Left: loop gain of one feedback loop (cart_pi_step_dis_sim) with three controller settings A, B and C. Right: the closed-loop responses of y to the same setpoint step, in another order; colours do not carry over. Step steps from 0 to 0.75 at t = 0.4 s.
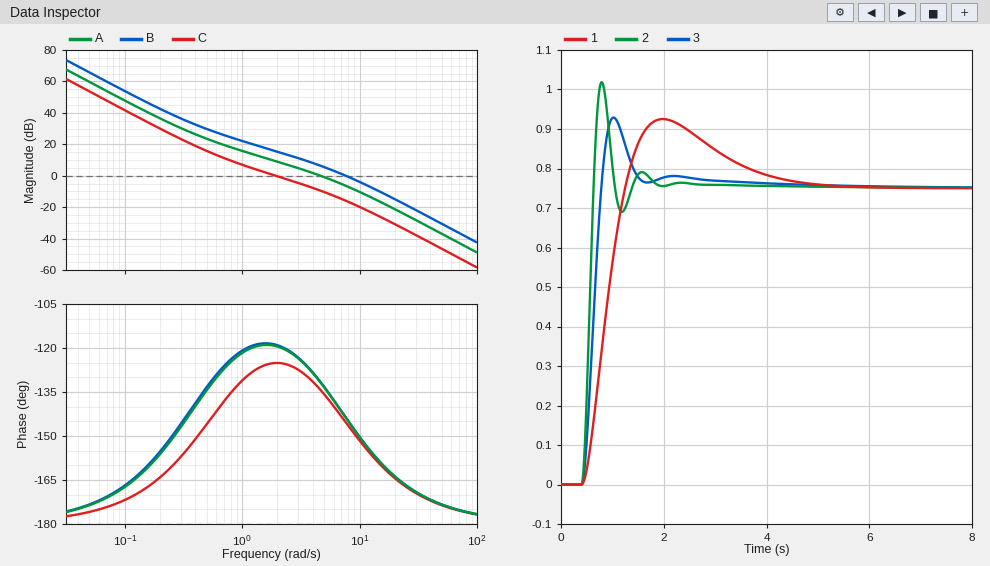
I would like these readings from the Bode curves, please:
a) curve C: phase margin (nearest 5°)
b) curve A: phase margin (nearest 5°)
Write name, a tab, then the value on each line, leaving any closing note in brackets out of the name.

curve C: phase margin	55°
curve A: phase margin	50°
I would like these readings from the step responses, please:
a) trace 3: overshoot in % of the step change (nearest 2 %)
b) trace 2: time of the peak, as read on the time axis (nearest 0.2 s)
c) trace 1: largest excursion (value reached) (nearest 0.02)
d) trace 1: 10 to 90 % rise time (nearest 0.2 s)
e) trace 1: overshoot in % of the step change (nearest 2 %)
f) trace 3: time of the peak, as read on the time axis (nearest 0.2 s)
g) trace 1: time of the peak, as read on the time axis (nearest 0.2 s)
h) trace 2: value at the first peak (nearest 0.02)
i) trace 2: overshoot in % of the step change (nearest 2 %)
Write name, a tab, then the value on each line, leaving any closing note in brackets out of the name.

trace 3: overshoot in % of the step change	24 %
trace 2: time of the peak, as read on the time axis	0.8 s
trace 1: largest excursion (value reached)	0.92
trace 1: 10 to 90 % rise time	0.6 s
trace 1: overshoot in % of the step change	24 %
trace 3: time of the peak, as read on the time axis	1.0 s
trace 1: time of the peak, as read on the time axis	2.0 s
trace 2: value at the first peak	1.02
trace 2: overshoot in % of the step change	36 %
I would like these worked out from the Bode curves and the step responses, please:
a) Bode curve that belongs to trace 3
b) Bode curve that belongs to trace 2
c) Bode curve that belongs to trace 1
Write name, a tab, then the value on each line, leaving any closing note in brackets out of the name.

Bode curve that belongs to trace 3	A
Bode curve that belongs to trace 2	B
Bode curve that belongs to trace 1	C
